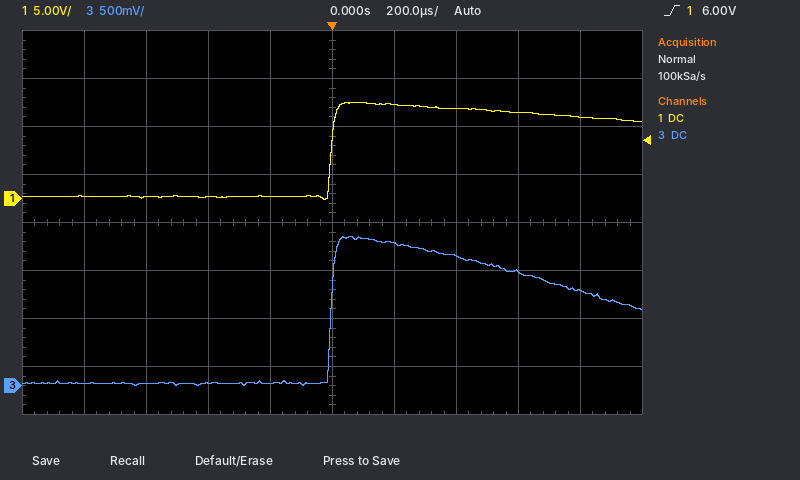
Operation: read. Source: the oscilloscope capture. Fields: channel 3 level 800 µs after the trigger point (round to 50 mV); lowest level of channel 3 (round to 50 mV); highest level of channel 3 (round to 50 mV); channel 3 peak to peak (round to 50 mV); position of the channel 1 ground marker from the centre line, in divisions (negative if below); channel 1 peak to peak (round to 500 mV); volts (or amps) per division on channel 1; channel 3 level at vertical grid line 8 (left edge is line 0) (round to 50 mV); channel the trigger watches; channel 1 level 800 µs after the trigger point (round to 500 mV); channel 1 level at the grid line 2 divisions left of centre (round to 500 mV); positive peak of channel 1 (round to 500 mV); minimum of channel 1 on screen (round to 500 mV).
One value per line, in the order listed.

1.00 V
0 mV
1.55 V
1.55 V
+0.5 div
10.0 V
5 V
1.20 V
channel 1
8.5 V
0.0 V
10.0 V
0.0 V
